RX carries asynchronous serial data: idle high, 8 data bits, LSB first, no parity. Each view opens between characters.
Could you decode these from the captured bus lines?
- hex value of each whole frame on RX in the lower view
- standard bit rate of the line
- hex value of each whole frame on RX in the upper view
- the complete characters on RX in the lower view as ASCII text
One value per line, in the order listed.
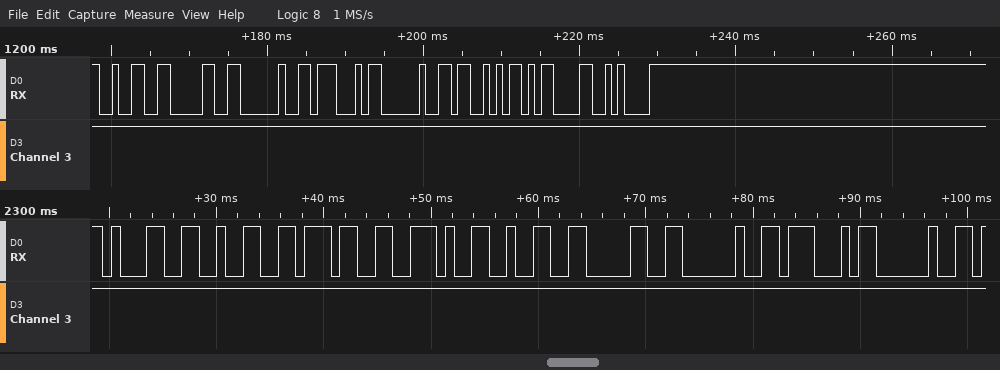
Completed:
31, 32, 37, 2E, 32, 30, 20, 47, 20
1200 baud
32, 30, 20, 47, 20, 53, 0D, 0A
"127.20 G "
